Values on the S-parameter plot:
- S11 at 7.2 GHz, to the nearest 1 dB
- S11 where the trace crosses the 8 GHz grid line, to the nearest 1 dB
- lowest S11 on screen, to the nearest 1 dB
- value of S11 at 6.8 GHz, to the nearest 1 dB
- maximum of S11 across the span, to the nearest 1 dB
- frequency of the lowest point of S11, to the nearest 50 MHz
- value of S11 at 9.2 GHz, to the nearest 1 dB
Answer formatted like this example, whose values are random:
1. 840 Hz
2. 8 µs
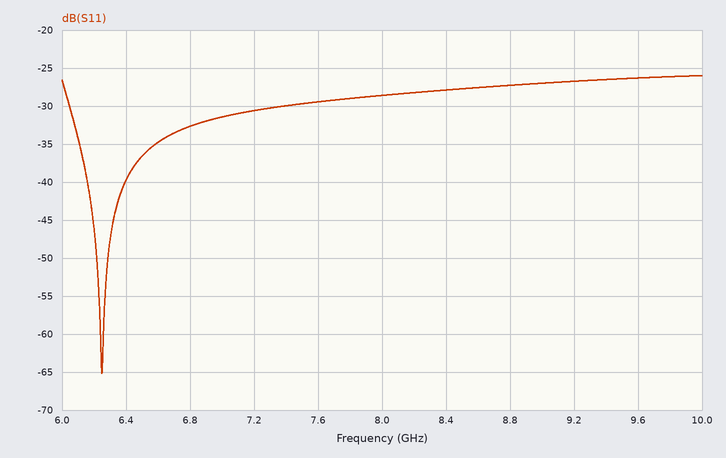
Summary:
1. -31 dB
2. -29 dB
3. -65 dB
4. -33 dB
5. -26 dB
6. 6.25 GHz
7. -27 dB
